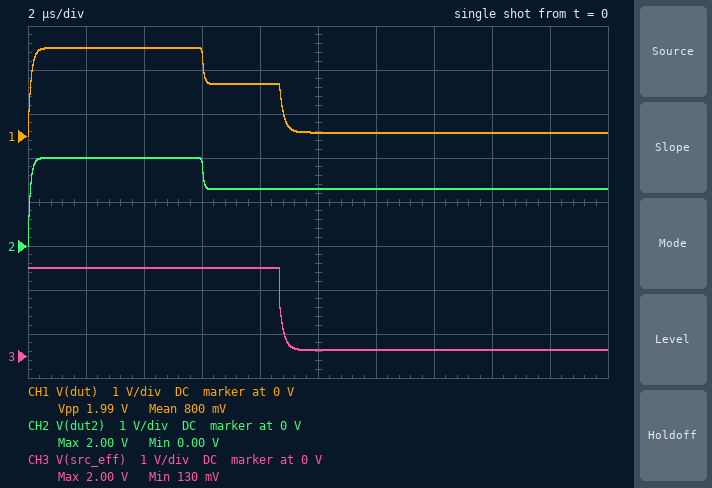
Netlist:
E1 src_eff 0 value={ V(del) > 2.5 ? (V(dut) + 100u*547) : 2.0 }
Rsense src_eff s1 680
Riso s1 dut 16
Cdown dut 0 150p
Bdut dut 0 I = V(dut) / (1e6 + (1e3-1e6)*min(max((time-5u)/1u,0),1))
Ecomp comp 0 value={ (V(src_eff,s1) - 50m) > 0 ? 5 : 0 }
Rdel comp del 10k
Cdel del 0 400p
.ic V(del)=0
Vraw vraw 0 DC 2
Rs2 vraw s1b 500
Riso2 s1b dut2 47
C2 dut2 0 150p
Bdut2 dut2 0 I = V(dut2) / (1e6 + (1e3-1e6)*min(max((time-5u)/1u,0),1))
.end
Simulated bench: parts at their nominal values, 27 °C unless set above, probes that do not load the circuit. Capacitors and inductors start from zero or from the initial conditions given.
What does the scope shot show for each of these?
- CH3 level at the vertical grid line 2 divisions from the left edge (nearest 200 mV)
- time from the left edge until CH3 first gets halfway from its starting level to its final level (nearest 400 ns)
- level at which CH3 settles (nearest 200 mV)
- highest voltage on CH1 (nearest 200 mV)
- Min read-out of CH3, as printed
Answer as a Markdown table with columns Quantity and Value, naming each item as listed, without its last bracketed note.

| Quantity | Value |
|---|---|
| CH3 level at the vertical grid line 2 divisions from the left edge | 2.0 V |
| time from the left edge until CH3 first gets halfway from its starting level to its final level | 8.8 µs |
| level at which CH3 settles | 200 mV |
| highest voltage on CH1 | 2.0 V |
| Min read-out of CH3, as printed | 130 mV |
